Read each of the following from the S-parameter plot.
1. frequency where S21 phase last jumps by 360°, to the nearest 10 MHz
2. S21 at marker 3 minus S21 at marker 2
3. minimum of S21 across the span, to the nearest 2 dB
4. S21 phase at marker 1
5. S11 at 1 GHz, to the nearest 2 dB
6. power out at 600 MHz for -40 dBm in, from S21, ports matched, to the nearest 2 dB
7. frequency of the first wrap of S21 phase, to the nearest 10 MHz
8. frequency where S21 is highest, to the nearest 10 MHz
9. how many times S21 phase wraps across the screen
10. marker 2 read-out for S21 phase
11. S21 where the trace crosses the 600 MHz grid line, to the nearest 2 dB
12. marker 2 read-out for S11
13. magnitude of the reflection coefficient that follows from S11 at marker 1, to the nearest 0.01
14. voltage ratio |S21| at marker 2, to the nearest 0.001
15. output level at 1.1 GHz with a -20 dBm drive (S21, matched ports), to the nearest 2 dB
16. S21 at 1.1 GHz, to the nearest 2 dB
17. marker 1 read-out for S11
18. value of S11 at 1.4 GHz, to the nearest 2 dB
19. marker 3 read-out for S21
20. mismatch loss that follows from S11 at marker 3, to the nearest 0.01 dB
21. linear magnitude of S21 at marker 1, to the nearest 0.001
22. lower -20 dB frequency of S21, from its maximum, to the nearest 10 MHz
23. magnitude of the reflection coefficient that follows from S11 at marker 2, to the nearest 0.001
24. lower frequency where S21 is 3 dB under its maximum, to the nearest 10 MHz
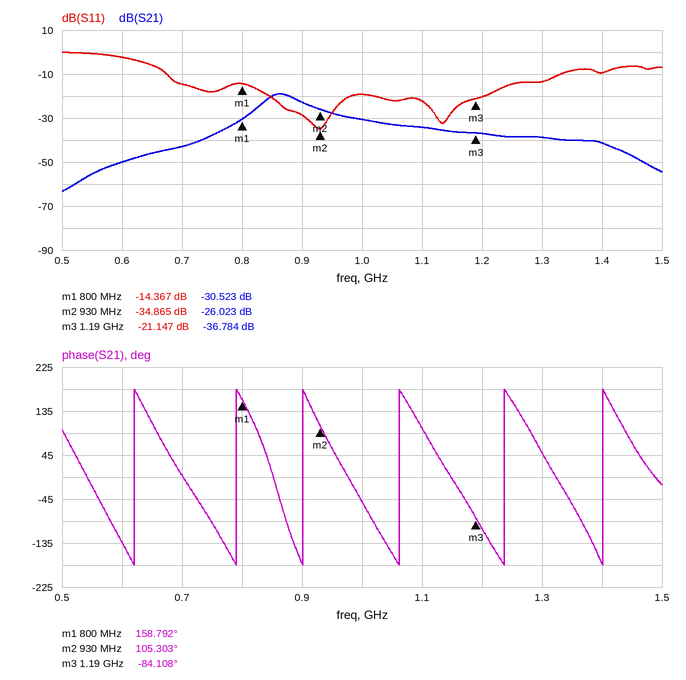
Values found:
1.40 GHz
-10.761 dB
-64 dB
158.792°
-20 dB
-90 dBm
620 MHz
860 MHz
6
105.303°
-50 dB
-34.865 dB
0.19
0.050
-54 dBm
-34 dB
-14.367 dB
-10 dB
-36.784 dB
0.03 dB
0.030
740 MHz
0.018
840 MHz
